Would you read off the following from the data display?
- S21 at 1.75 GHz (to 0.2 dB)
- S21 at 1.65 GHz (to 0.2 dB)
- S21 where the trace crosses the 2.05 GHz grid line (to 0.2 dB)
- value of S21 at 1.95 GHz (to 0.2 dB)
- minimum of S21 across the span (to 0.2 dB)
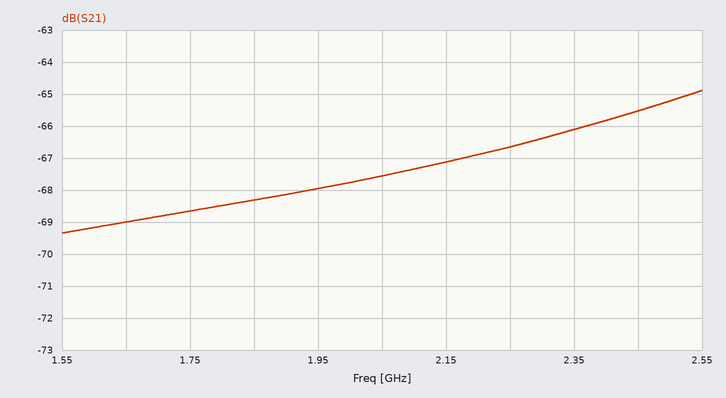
-68.6 dB
-69.0 dB
-67.6 dB
-68.0 dB
-69.4 dB
